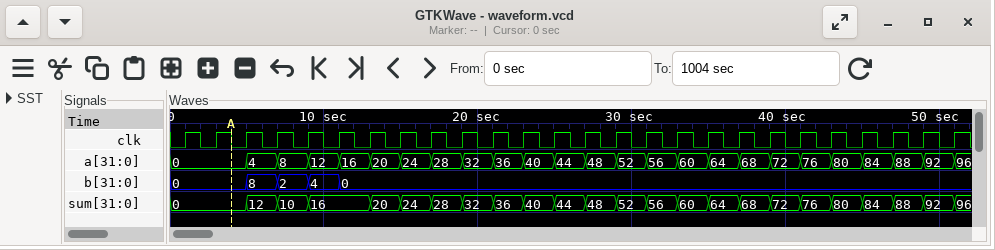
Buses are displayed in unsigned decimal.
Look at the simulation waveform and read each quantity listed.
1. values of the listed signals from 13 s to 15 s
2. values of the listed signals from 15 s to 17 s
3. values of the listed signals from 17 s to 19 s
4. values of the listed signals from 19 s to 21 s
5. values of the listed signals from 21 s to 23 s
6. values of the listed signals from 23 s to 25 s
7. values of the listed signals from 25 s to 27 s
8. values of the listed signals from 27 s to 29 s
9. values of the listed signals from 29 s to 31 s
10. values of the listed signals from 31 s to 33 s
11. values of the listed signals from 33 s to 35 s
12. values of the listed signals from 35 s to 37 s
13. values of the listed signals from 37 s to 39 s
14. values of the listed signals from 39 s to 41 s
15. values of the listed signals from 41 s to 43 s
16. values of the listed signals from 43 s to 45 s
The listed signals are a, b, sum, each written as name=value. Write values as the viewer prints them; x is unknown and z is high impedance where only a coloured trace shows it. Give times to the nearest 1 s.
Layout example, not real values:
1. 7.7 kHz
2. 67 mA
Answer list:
1. a=20, b=0, sum=20
2. a=24, b=0, sum=24
3. a=28, b=0, sum=28
4. a=32, b=0, sum=32
5. a=36, b=0, sum=36
6. a=40, b=0, sum=40
7. a=44, b=0, sum=44
8. a=48, b=0, sum=48
9. a=52, b=0, sum=52
10. a=56, b=0, sum=56
11. a=60, b=0, sum=60
12. a=64, b=0, sum=64
13. a=68, b=0, sum=68
14. a=72, b=0, sum=72
15. a=76, b=0, sum=76
16. a=80, b=0, sum=80
